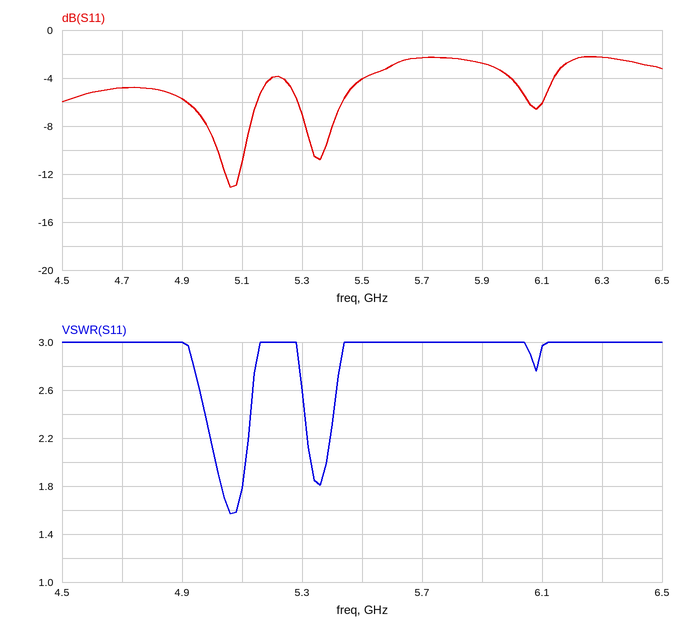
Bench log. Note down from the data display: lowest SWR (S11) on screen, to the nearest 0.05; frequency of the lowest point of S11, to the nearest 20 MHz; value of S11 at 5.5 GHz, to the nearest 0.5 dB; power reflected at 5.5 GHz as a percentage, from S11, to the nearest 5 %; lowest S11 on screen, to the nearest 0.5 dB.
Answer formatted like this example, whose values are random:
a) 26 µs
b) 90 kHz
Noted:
a) 1.55
b) 5.06 GHz
c) -4.0 dB
d) 40 %
e) -13.0 dB
